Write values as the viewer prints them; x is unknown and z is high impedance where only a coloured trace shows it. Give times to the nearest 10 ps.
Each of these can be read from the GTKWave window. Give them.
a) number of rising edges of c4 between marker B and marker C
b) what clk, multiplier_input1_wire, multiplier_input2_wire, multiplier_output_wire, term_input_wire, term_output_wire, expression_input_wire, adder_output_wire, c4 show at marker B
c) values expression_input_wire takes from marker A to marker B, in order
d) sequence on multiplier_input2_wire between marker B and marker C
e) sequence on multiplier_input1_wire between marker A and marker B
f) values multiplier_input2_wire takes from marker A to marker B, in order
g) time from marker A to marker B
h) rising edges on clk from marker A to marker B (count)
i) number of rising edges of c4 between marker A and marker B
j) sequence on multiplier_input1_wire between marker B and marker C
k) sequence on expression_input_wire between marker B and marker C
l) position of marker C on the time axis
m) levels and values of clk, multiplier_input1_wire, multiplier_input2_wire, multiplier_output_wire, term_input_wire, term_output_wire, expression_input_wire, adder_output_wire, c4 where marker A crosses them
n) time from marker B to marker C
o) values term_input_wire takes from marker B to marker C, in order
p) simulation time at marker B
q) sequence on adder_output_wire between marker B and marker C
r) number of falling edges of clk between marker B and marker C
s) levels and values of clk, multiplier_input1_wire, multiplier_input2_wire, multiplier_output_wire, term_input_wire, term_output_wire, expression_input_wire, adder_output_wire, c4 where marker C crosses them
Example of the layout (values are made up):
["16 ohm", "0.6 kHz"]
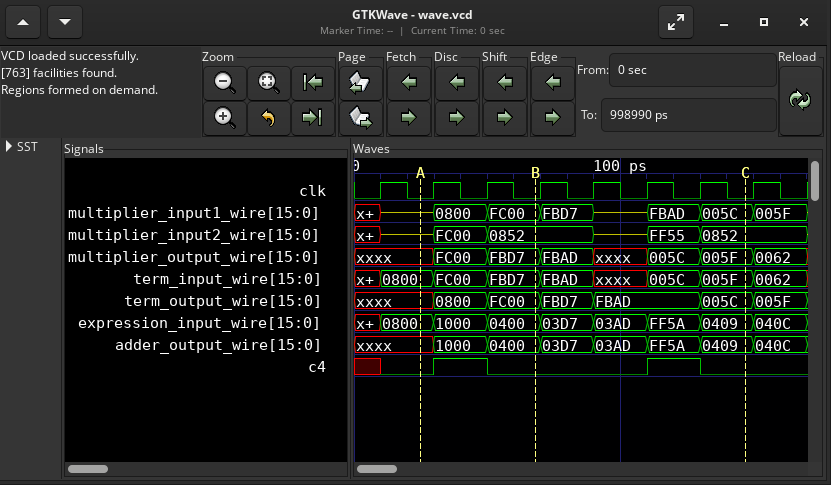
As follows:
["1", "clk=0, multiplier_input1_wire=FC00, multiplier_input2_wire=0852, multiplier_output_wire=FBD7, term_input_wire=FBD7, term_output_wire=FC00, expression_input_wire=0400, adder_output_wire=0400, c4=0", "0800, 1000, 0400", "0852, z, FF55, 0852", "z, 0800, FC00", "z, FC00, 0852", "40 ps", "2", "1", "FC00, FBD7, z, FBAD, 005C", "0400, 03D7, 03AD, FF5A, 0409", "150 ps", "clk=0, multiplier_input1_wire=z, multiplier_input2_wire=z, multiplier_output_wire=xxxx, term_input_wire=0800, term_output_wire=xxxx, expression_input_wire=0800, adder_output_wire=xxxx, c4=0", "80 ps", "FBD7, FBAD, xxxx, 005C, 005F", "70 ps", "0400, 03D7, 03AD, FF5A, 0409", "4", "clk=0, multiplier_input1_wire=005C, multiplier_input2_wire=0852, multiplier_output_wire=005F, term_input_wire=005F, term_output_wire=005C, expression_input_wire=0409, adder_output_wire=0409, c4=0"]
